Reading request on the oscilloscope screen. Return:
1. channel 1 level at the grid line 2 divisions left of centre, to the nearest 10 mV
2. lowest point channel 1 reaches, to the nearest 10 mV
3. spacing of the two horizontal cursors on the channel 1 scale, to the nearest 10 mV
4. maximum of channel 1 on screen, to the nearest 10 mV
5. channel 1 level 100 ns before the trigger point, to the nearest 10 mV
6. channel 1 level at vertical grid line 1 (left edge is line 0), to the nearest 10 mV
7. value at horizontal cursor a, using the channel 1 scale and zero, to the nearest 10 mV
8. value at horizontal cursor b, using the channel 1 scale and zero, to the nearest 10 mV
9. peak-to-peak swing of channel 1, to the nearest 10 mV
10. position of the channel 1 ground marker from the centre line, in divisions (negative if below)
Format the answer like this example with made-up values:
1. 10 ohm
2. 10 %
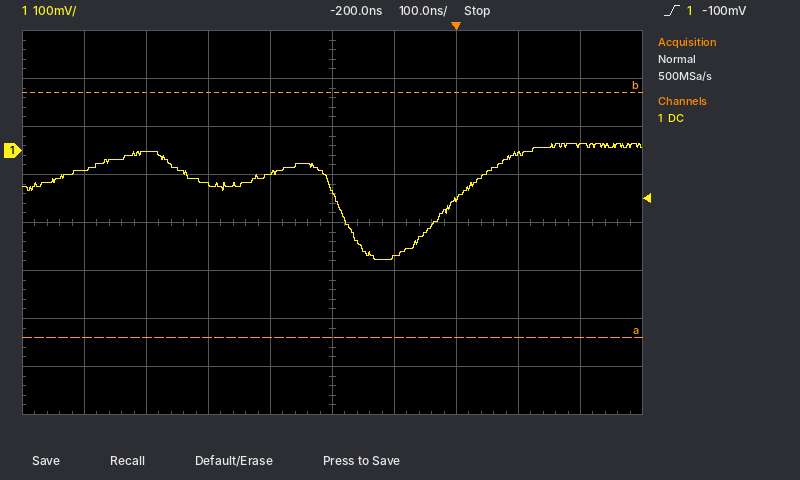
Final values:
1. -70 mV
2. -230 mV
3. 510 mV
4. 10 mV
5. -220 mV
6. -40 mV
7. -390 mV
8. 120 mV
9. 240 mV
10. +1.5 div
